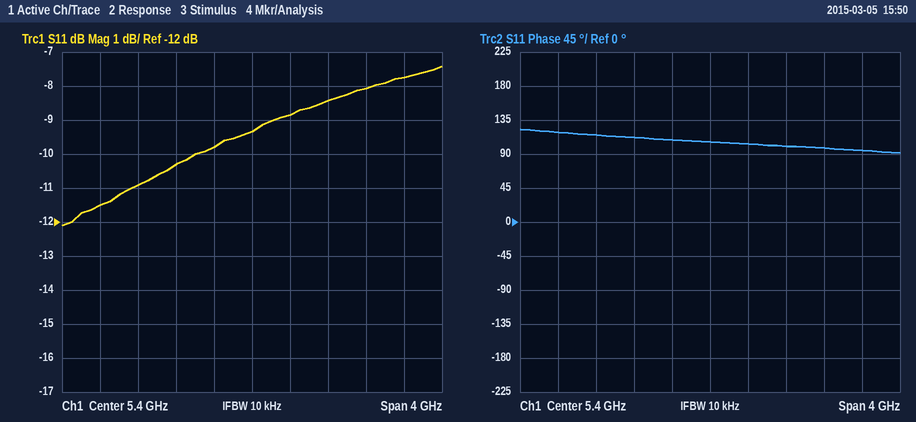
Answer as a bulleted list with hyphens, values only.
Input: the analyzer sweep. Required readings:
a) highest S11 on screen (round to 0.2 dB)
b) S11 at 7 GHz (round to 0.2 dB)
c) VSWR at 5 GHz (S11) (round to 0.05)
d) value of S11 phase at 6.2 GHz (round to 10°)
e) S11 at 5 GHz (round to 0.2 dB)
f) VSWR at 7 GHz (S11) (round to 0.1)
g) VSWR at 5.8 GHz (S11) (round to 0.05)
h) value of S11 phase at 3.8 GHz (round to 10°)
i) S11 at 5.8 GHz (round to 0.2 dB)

- -7.4 dB
- -7.8 dB
- 1.95
- 100°
- -9.8 dB
- 2.4
- 2.15
- 120°
- -8.8 dB
